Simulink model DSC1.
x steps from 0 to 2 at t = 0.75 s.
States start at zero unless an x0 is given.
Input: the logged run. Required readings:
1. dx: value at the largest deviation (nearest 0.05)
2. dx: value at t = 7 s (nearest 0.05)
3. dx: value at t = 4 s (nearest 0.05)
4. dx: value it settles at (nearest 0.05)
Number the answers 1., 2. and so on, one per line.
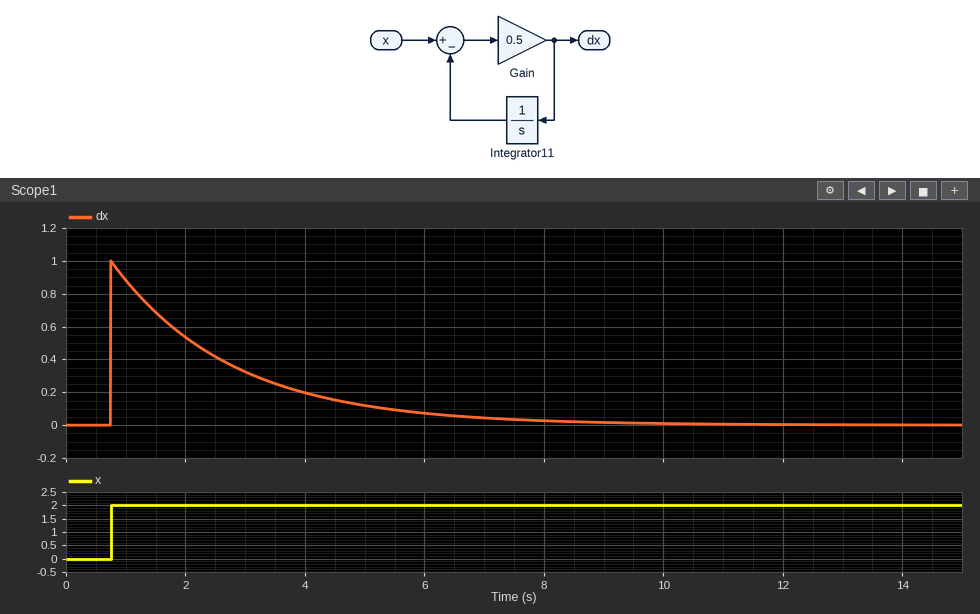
1. 1.00
2. 0.05
3. 0.20
4. 0.00
